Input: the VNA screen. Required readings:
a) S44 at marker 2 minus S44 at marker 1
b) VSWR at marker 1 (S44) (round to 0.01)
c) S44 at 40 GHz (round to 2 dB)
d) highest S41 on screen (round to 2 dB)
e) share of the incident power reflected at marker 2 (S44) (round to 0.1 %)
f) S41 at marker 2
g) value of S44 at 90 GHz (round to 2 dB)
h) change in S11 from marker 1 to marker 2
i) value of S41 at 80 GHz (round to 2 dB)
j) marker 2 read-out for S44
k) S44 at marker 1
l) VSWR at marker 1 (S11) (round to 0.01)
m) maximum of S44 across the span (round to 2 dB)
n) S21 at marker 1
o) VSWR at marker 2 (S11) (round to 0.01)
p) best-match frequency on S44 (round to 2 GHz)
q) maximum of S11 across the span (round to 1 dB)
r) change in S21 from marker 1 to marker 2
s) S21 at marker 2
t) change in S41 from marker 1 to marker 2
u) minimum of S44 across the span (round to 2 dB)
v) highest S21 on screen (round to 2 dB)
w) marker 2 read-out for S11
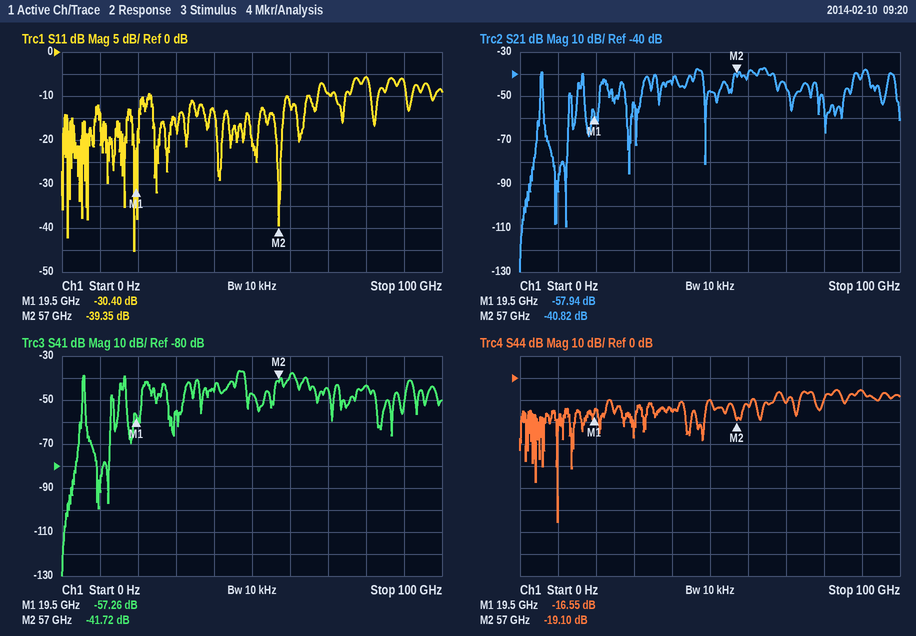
-2.55 dB
1.35
-14 dB
-36 dB
1.2 %
-41.72 dB
-6 dB
-8.95 dB
-44 dB
-19.10 dB
-16.55 dB
1.06
-6 dB
-57.94 dB
1.02
10 GHz
-6 dB
17.12 dB
-40.82 dB
15.54 dB
-66 dB
-38 dB
-39.35 dB
